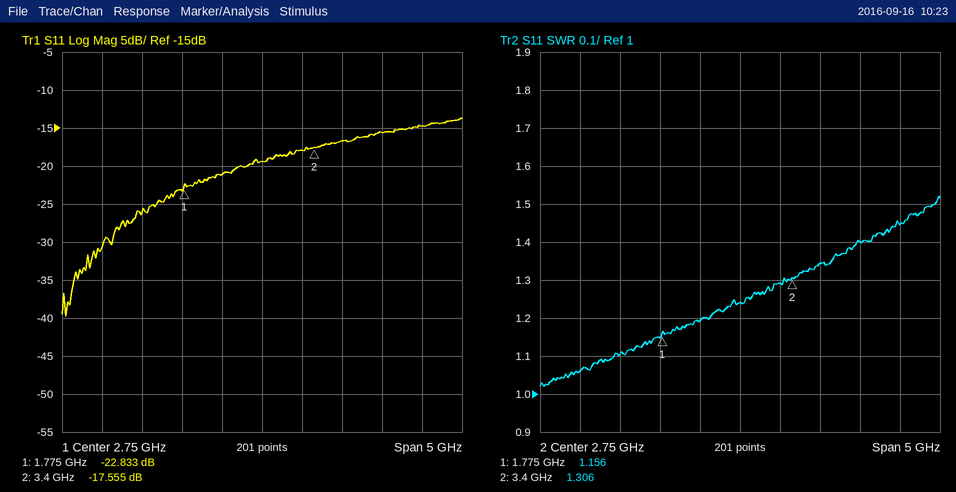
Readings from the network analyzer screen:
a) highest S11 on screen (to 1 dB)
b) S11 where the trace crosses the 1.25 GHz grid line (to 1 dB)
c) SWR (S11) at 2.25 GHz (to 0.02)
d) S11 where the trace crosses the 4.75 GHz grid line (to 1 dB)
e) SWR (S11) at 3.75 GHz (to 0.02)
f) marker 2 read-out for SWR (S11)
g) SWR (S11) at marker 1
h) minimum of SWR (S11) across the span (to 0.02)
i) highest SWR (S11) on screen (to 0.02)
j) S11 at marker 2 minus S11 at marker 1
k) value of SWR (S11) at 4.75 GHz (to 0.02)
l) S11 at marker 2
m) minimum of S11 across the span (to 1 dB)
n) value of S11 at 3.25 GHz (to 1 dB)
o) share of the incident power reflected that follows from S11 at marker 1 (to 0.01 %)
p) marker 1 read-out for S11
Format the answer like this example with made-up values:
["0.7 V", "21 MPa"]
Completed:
["-14 dB", "-26 dB", "1.20", "-15 dB", "1.34", "1.306", "1.156", "1.02", "1.52", "5.278 dB", "1.44", "-17.555 dB", "-40 dB", "-18 dB", "0.52 %", "-22.833 dB"]
